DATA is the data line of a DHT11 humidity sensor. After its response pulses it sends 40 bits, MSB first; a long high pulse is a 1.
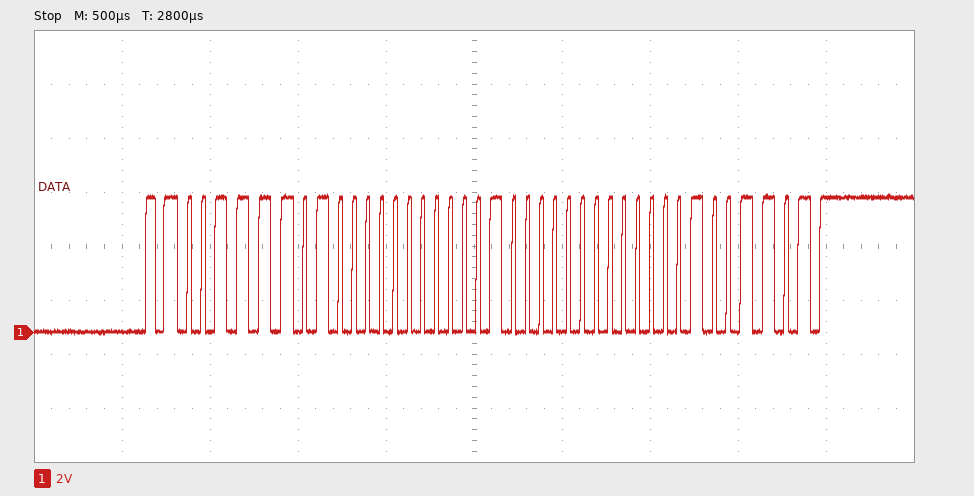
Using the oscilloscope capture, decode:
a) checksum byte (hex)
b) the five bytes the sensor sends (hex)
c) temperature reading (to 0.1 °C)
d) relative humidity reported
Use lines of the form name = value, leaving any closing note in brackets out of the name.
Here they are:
checksum byte = 0x4D
the five bytes the sensor sends = 3D 00 10 00 4D
temperature reading = 16.0 °C
relative humidity reported = 61 %
